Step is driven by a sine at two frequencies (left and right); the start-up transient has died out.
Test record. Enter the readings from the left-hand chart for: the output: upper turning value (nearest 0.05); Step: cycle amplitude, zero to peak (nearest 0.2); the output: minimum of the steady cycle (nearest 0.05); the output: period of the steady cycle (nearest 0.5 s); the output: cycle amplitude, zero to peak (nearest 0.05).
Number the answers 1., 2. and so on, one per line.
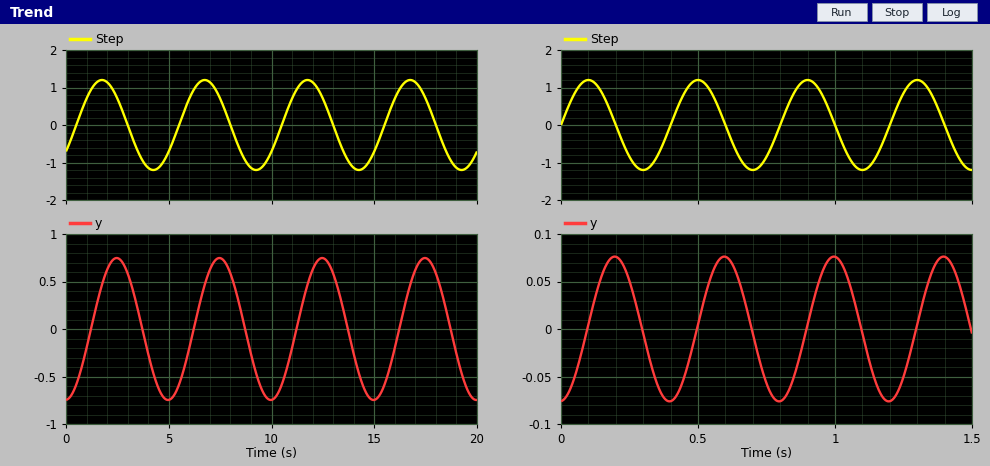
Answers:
1. 0.75
2. 1.2
3. -0.75
4. 5.0 s
5. 0.75
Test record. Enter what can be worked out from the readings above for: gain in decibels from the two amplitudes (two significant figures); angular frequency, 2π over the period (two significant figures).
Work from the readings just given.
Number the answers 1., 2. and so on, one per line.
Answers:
1. -4.1 dB
2. 1.3 rad/s
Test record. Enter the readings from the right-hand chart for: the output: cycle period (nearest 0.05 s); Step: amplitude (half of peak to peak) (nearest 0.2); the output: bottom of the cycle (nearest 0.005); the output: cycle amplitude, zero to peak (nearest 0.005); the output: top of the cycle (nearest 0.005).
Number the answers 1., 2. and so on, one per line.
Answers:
1. 0.40 s
2. 1.2
3. -0.075
4. 0.075
5. 0.075
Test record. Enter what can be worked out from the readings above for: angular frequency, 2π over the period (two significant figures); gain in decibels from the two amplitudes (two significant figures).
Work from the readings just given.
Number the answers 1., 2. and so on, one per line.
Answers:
1. 16 rad/s
2. -24 dB
